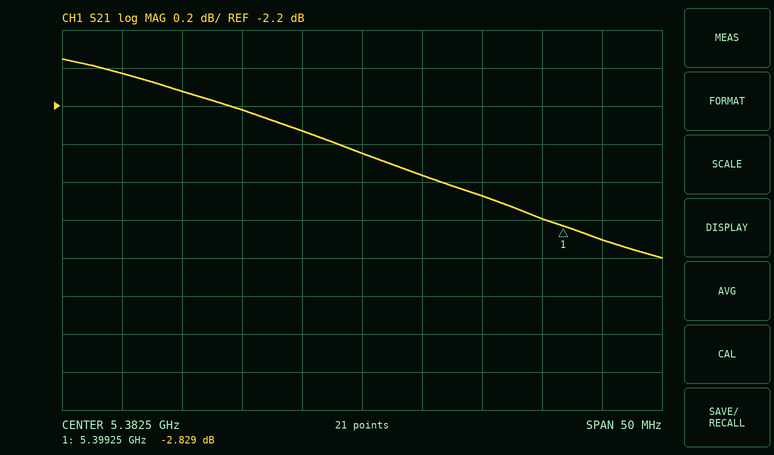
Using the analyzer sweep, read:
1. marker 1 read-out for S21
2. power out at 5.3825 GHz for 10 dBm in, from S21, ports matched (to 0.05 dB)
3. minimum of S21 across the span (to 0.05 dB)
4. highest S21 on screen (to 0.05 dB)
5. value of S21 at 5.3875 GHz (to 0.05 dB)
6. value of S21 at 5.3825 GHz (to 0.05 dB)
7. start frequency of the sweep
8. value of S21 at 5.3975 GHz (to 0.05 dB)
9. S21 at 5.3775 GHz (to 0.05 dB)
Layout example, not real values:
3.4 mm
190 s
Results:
-2.829 dB
7.55 dBm
-3.00 dB
-1.95 dB
-2.55 dB
-2.45 dB
5.3575 GHz
-2.80 dB
-2.35 dB
